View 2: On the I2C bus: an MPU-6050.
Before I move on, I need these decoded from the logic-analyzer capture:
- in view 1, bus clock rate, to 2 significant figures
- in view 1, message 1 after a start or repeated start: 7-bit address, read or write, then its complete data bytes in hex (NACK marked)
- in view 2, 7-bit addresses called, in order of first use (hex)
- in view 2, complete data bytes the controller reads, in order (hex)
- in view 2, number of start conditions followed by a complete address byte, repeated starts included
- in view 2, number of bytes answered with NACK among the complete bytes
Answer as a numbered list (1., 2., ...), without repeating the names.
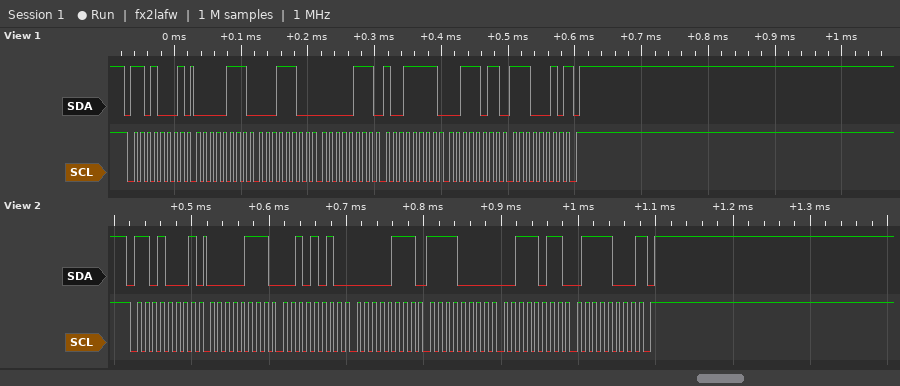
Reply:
1. 100 kHz
2. 0x68 read: 07 1C 07 9F 3B E2 NACK
3. 0x68
4. 07 2A 07 F0 3B 78
5. 1
6. 1
